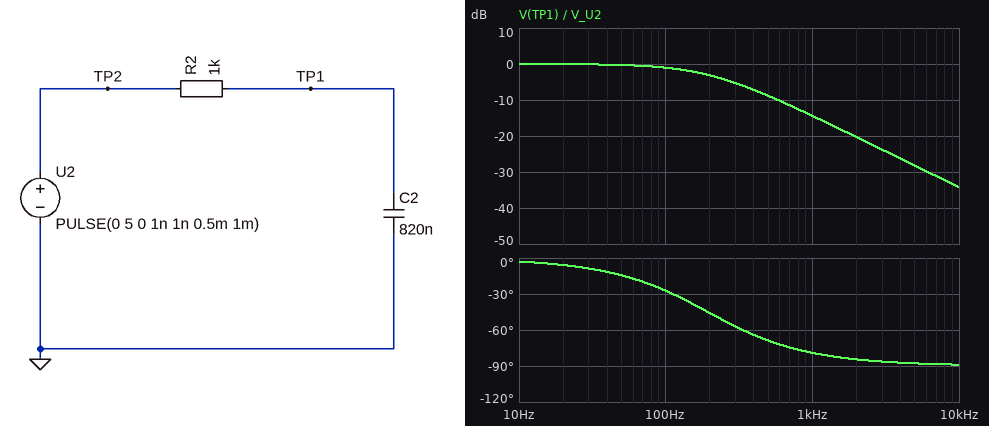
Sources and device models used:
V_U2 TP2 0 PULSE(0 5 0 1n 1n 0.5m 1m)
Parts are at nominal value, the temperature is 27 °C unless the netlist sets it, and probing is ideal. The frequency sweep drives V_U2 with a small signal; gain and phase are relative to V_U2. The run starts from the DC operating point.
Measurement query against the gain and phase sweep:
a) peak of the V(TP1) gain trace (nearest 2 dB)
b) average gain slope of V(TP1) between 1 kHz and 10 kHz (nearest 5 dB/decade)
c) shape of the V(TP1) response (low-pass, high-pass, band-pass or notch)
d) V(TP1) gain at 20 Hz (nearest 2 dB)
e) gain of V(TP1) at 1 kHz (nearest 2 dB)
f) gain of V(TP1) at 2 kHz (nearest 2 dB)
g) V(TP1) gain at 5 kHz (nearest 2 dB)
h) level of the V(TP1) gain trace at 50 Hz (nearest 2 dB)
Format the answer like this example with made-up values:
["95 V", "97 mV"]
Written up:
["0 dB", "-20 dB/decade", "low-pass", "0 dB", "-14 dB", "-20 dB", "-28 dB", "0 dB"]
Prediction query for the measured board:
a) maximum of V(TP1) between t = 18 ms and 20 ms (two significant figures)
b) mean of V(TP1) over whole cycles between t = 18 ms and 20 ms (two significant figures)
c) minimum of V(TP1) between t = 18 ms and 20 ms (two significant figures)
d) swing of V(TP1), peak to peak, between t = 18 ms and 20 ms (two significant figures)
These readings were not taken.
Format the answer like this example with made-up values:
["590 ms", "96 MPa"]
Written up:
["3.2 V", "2.5 V", "1.8 V", "1.5 V"]
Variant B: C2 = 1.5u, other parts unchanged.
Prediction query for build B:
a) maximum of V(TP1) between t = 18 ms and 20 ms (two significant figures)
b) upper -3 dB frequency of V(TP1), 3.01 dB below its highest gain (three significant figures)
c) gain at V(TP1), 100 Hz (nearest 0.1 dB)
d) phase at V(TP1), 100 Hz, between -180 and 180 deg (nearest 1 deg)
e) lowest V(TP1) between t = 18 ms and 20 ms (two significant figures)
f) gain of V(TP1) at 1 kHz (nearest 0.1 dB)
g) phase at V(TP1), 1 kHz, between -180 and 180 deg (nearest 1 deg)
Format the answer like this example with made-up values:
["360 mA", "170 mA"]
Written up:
["2.9 V", "106 Hz", "-2.8 dB", "-43 deg", "2.1 V", "-19.5 dB", "-84 deg"]
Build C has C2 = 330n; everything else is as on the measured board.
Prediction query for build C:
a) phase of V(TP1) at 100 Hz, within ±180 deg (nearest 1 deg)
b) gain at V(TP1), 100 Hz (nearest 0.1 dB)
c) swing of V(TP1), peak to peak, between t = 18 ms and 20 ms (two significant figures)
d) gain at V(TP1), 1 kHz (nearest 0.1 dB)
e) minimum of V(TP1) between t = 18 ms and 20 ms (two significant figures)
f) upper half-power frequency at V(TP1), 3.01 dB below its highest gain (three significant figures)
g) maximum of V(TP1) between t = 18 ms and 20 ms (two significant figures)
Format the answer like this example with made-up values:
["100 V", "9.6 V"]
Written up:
["-12 deg", "-0.2 dB", "3.2 V", "-7.2 dB", "900 mV", "482 Hz", "4.1 V"]
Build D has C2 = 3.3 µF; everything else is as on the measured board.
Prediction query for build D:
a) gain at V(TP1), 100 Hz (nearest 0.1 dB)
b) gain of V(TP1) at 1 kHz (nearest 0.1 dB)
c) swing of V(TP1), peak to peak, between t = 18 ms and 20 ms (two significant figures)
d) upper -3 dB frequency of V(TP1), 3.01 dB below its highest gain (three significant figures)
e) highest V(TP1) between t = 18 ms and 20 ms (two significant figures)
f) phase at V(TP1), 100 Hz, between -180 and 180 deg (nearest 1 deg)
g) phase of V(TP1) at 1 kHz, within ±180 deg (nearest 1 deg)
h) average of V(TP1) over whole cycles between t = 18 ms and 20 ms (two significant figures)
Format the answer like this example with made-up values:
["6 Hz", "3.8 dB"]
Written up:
["-7.2 dB", "-26.3 dB", "380 mV", "48.2 Hz", "2.7 V", "-64 deg", "-87 deg", "2.5 V"]
